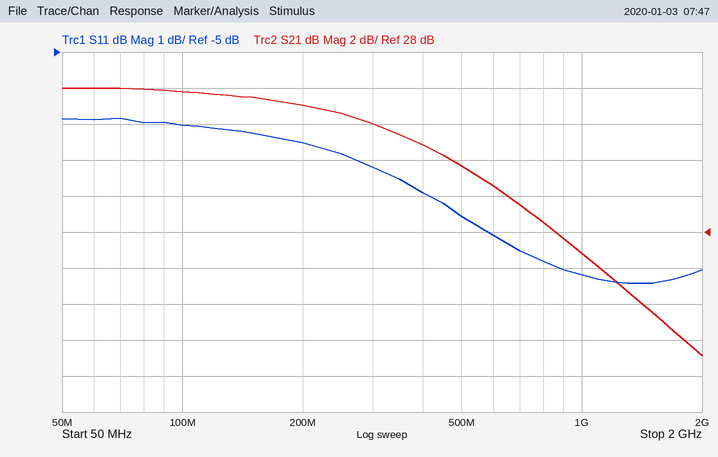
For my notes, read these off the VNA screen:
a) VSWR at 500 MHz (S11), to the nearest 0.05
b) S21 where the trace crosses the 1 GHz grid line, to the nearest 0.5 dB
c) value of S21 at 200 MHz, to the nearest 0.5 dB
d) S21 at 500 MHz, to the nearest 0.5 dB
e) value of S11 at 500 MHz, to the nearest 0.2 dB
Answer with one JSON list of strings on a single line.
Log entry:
["2.00", "27.0 dB", "35.0 dB", "31.5 dB", "-9.6 dB"]
